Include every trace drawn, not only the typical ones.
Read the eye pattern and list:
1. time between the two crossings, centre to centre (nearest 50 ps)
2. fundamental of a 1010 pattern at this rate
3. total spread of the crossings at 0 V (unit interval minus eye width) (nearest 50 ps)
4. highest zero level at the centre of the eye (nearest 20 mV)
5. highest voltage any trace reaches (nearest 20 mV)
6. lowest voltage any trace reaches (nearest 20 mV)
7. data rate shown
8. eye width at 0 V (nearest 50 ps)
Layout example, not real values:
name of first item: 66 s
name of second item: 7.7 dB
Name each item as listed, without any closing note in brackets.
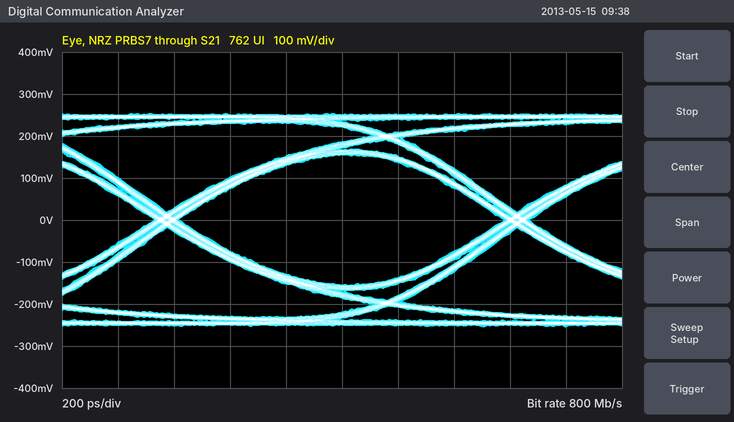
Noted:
time between the two crossings, centre to centre: 1.25 ns
fundamental of a 1010 pattern at this rate: 400 MHz
total spread of the crossings at 0 V (unit interval minus eye width): 100 ps
highest zero level at the centre of the eye: -160 mV
highest voltage any trace reaches: 260 mV
lowest voltage any trace reaches: -260 mV
data rate shown: 800 Mb/s
eye width at 0 V: 1.15 ns
